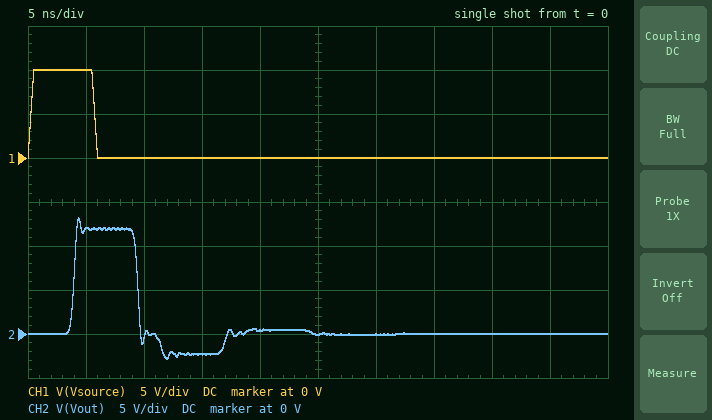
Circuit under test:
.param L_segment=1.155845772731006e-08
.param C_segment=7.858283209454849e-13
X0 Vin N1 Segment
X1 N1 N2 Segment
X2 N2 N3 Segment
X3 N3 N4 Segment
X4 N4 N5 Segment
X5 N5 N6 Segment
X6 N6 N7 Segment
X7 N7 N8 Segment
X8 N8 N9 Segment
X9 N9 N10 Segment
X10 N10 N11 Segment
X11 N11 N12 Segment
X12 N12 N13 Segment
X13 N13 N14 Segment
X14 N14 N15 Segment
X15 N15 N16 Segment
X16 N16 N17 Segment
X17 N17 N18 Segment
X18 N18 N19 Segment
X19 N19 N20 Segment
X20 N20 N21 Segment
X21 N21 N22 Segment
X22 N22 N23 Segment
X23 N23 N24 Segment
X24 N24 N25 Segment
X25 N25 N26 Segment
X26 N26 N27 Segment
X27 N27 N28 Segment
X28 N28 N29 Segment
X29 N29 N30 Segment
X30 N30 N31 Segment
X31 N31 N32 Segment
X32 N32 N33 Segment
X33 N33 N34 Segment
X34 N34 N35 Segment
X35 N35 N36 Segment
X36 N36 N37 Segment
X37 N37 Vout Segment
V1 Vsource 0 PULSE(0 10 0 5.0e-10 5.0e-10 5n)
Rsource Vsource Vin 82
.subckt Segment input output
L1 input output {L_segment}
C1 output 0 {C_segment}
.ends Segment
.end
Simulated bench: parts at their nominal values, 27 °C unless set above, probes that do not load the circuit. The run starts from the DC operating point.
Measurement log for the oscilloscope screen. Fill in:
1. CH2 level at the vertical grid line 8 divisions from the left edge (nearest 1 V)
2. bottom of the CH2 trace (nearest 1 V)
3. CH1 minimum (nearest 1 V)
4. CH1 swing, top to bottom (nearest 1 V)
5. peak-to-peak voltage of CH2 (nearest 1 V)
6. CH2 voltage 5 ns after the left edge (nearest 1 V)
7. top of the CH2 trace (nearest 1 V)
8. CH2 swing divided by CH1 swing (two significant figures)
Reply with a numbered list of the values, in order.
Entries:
1. 0 V
2. -3 V
3. 0 V
4. 10 V
5. 16 V
6. 12 V
7. 13 V
8. 1.6
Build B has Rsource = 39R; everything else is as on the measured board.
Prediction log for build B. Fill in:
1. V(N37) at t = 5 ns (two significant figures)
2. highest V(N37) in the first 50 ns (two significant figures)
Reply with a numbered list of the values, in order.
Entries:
1. 15 V
2. 16 V
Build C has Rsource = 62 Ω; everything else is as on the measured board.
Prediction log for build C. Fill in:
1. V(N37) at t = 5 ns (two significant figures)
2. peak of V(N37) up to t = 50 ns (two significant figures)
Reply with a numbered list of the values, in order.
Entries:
1. 13 V
2. 14 V
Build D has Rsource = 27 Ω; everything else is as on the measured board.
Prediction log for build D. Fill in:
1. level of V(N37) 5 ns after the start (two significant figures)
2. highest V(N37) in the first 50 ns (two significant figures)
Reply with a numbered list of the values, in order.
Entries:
1. 16 V
2. 17 V
